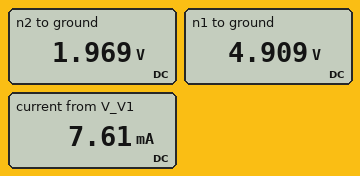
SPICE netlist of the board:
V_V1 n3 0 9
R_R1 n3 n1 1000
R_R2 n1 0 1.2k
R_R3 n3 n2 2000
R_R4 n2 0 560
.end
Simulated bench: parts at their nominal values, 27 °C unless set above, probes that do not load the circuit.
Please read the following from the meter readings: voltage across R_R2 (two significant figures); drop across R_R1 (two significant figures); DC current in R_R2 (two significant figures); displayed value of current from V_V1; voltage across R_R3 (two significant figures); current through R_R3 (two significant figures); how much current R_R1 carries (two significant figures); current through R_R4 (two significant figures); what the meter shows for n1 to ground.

4.9 V
4.1 V
4.1 mA
7.61 mA
7.0 V
3.5 mA
4.1 mA
3.5 mA
4.909 V
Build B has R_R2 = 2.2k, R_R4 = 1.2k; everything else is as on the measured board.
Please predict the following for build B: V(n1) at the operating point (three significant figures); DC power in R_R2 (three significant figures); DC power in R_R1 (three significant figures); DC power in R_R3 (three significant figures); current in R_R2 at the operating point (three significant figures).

6.19 V
17.4 mW
7.91 mW
15.8 mW
2.81 mA
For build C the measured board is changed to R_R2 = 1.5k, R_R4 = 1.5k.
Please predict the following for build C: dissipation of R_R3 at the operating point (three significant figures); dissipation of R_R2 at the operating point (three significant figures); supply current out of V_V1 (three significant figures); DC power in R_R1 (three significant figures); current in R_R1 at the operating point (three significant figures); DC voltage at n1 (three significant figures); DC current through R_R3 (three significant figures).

13.2 mW
19.4 mW
6.17 mA
13.0 mW
3.60 mA
5.40 V
2.57 mA
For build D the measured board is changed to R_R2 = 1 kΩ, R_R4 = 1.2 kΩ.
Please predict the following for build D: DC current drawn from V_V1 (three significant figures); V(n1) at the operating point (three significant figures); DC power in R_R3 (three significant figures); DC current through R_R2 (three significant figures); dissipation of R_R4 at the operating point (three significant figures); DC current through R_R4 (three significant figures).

7.31 mA
4.50 V
15.8 mW
4.50 mA
9.49 mW
2.81 mA
